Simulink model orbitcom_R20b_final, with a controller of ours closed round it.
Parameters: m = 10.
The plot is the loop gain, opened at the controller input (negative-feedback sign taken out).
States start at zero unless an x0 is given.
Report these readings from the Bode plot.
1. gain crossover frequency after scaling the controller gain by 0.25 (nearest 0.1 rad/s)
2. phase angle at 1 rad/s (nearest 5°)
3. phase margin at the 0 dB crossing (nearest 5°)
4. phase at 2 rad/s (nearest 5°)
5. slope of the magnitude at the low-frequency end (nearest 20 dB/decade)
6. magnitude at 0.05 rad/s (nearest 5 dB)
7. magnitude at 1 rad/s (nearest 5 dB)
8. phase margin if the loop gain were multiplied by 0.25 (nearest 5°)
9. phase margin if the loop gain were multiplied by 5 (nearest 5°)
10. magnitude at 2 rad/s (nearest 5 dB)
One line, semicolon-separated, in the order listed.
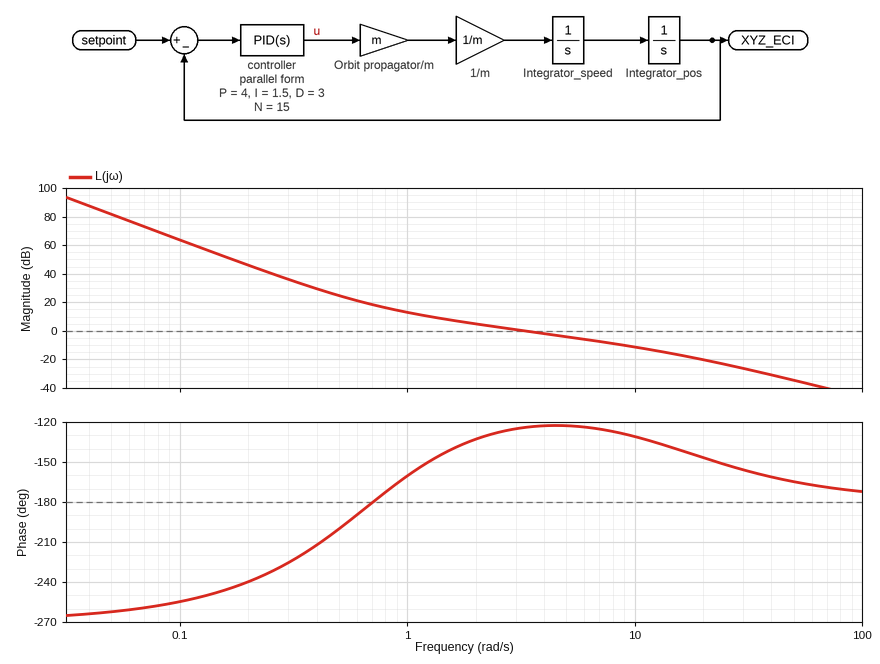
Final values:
1.1 rad/s; -160°; 55°; -135°; -60 dB/decade; 80 dB; 15 dB; 25°; 45°; 5 dB
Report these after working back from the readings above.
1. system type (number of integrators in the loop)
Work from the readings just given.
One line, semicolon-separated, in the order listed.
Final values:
3
